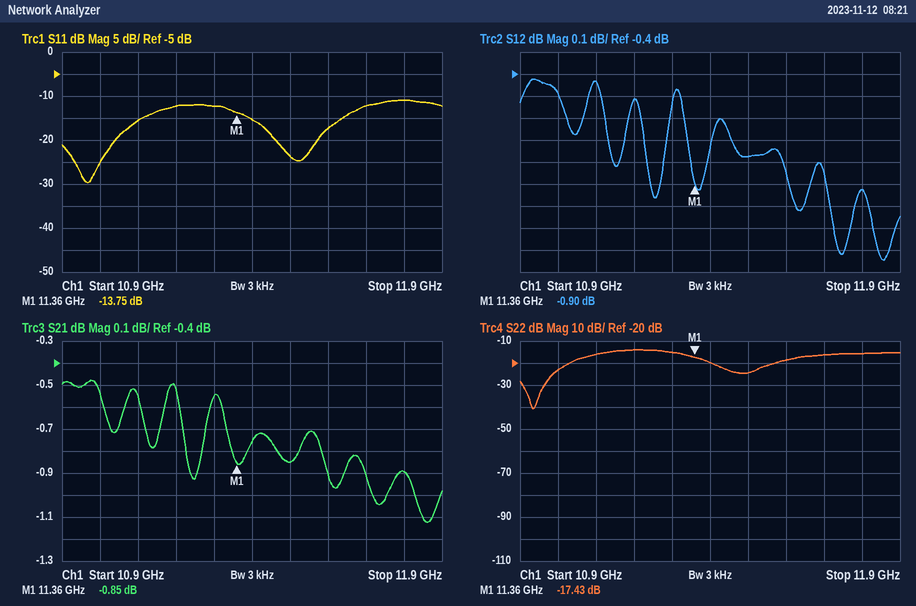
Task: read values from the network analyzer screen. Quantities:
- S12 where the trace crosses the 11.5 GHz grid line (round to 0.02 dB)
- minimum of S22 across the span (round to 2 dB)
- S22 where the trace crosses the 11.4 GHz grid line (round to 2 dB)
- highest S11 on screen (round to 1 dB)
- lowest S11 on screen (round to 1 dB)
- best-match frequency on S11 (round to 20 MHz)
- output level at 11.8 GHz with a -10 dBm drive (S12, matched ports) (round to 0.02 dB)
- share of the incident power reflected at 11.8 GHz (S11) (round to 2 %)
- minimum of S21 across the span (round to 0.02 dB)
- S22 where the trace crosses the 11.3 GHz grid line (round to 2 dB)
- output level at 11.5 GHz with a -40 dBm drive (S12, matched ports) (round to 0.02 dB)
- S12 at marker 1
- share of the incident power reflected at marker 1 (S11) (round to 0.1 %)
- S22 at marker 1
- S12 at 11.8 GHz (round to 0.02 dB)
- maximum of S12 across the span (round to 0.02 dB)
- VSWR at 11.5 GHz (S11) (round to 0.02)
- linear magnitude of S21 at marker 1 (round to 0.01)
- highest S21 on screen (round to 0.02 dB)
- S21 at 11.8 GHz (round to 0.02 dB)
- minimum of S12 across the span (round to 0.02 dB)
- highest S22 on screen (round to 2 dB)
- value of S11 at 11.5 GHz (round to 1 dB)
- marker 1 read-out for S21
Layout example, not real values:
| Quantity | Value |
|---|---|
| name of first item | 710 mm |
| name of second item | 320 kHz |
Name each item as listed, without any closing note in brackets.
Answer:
| Quantity | Value |
|---|---|
| S12 where the trace crosses the 11.5 GHz grid line | -0.78 dB |
| minimum of S22 across the span | -40 dB |
| S22 where the trace crosses the 11.4 GHz grid line | -20 dB |
| highest S11 on screen | -11 dB |
| lowest S11 on screen | -30 dB |
| best-match frequency on S11 | 10.96 GHz |
| output level at 11.8 GHz with a -10 dBm drive (S12, matched ports) | -10.92 dBm |
| share of the incident power reflected at 11.8 GHz (S11) | 8 % |
| minimum of S21 across the span | -1.12 dB |
| S22 where the trace crosses the 11.3 GHz grid line | -16 dB |
| output level at 11.5 GHz with a -40 dBm drive (S12, matched ports) | -40.78 dBm |
| S12 at marker 1 | -0.90 dB |
| share of the incident power reflected at marker 1 (S11) | 4.2 % |
| S22 at marker 1 | -17.43 dB |
| S12 at 11.8 GHz | -0.92 dB |
| maximum of S12 across the span | -0.42 dB |
| VSWR at 11.5 GHz (S11) | 1.14 |
| linear magnitude of S21 at marker 1 | 0.91 |
| highest S21 on screen | -0.48 dB |
| S21 at 11.8 GHz | -0.90 dB |
| minimum of S12 across the span | -1.24 dB |
| highest S22 on screen | -14 dB |
| value of S11 at 11.5 GHz | -24 dB |
| marker 1 read-out for S21 | -0.85 dB |
